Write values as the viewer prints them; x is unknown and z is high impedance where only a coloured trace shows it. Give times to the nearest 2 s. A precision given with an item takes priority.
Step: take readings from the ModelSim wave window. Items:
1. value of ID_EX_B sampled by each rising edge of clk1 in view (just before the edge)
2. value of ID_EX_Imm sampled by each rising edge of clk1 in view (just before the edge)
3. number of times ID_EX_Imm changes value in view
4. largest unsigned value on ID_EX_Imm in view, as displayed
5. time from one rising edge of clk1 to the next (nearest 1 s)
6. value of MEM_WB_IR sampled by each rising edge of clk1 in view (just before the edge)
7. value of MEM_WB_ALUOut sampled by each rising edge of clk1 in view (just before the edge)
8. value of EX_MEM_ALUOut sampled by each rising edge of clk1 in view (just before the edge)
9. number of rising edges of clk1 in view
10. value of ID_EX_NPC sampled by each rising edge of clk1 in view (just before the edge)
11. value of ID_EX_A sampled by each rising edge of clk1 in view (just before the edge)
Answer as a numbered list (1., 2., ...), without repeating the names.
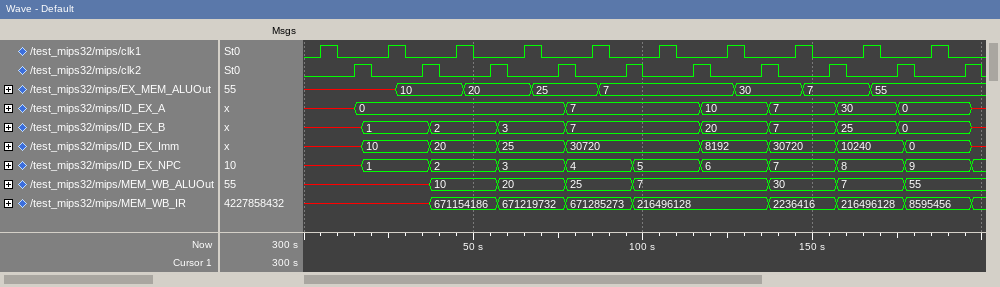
1. x, 1, 2, 3, 7, 7, 20, 7, 25, 0
2. x, 10, 20, 25, 30720, 30720, 8192, 30720, 10240, 0
3. 9
4. 30720
5. 20 s
6. x, x, 671154186, 671219732, 671285273, 216496128, 216496128, 2236416, 216496128, 8595456
7. x, x, 10, 20, 25, 7, 7, 30, 7, 55
8. x, x, 10, 20, 25, 7, 7, 30, 7, 55
9. 10
10. x, 1, 2, 3, 4, 5, 6, 7, 8, 9
11. x, 0, 0, 0, 7, 7, 10, 7, 30, 0
